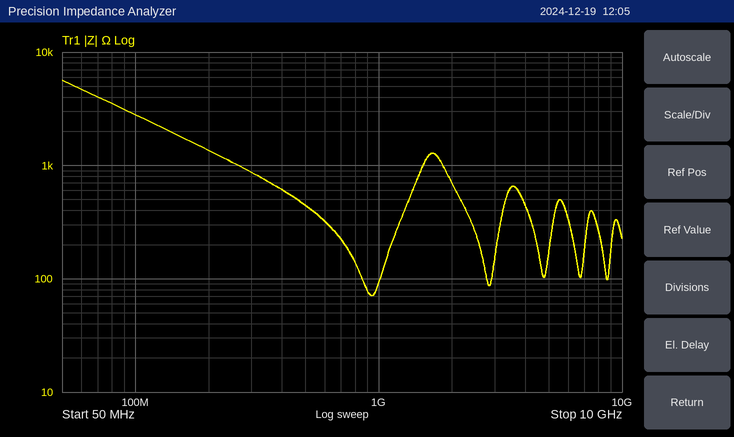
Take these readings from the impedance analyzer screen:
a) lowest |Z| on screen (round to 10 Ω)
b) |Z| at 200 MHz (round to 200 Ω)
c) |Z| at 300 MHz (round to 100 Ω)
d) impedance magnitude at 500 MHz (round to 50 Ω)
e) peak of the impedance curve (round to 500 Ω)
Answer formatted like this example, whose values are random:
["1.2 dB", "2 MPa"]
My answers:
["70 Ω", "1.4 kΩ", "900 Ω", "450 Ω", "5.5 kΩ"]
